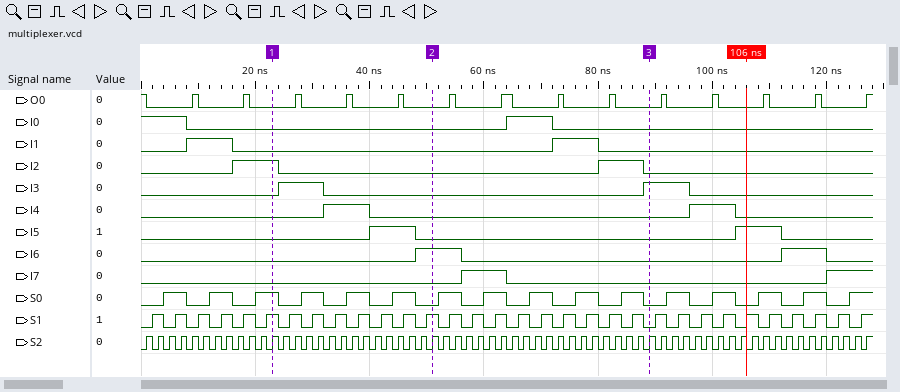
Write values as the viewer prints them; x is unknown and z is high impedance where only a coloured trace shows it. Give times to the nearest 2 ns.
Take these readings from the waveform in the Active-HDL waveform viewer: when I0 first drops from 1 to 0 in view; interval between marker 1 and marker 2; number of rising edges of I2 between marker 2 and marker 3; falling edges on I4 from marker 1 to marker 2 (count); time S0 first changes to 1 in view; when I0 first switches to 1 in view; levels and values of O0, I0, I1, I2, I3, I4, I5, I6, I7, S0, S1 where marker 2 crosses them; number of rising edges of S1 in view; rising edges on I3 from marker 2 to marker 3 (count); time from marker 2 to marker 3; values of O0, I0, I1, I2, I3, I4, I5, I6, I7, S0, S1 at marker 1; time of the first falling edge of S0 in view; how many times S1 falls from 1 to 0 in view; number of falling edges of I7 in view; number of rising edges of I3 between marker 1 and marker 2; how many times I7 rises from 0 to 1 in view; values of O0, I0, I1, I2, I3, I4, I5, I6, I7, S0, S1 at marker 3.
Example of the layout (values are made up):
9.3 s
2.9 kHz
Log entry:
8 ns
28 ns
1
1
4 ns
64 ns
O0=0, I0=0, I1=0, I2=0, I3=0, I4=0, I5=0, I6=1, I7=0, S0=0, S1=1
32
1
38 ns
O0=0, I0=0, I1=0, I2=1, I3=0, I4=0, I5=0, I6=0, I7=0, S0=1, S1=1
8 ns
31
1
1
2
O0=0, I0=0, I1=0, I2=0, I3=1, I4=0, I5=0, I6=0, I7=0, S0=0, S1=0
